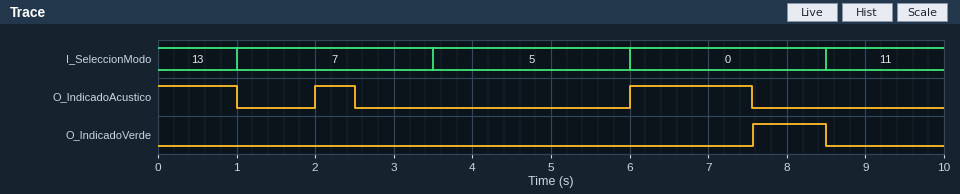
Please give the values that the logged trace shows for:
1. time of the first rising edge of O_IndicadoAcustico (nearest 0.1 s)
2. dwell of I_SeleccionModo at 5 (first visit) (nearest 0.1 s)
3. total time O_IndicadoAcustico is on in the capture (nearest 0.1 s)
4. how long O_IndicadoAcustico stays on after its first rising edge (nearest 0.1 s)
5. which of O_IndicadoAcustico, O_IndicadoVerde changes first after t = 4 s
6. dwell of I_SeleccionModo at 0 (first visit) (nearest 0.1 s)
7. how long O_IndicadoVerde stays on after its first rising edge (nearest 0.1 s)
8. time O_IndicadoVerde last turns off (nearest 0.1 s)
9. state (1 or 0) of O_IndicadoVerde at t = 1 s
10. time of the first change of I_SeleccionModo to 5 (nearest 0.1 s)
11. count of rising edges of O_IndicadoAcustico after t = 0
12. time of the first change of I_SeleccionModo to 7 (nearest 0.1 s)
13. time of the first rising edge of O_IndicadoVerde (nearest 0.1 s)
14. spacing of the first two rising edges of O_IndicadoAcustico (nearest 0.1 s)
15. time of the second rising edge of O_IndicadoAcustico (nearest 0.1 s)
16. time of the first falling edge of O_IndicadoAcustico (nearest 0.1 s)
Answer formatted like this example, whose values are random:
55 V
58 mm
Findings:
2.0 s
2.5 s
3.1 s
0.5 s
O_IndicadoAcustico
2.5 s
0.9 s
8.5 s
0
3.5 s
2
1.0 s
7.6 s
4.0 s
6.0 s
1.0 s
